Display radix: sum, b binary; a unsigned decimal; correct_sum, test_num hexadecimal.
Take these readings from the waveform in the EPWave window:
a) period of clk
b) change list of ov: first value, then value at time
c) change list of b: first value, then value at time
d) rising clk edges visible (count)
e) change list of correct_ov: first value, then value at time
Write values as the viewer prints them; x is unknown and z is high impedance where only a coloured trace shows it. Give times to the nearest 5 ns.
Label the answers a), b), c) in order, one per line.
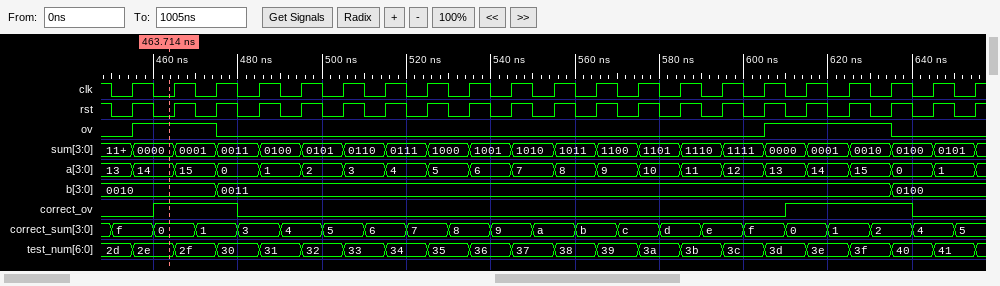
a) 10 ns
b) 0, 1 at 455 ns, 0 at 475 ns, 1 at 605 ns, 0 at 635 ns
c) 0010, 0011 at 475 ns, 0100 at 635 ns
d) 21
e) 0, 1 at 460 ns, 0 at 480 ns, 1 at 610 ns, 0 at 640 ns
